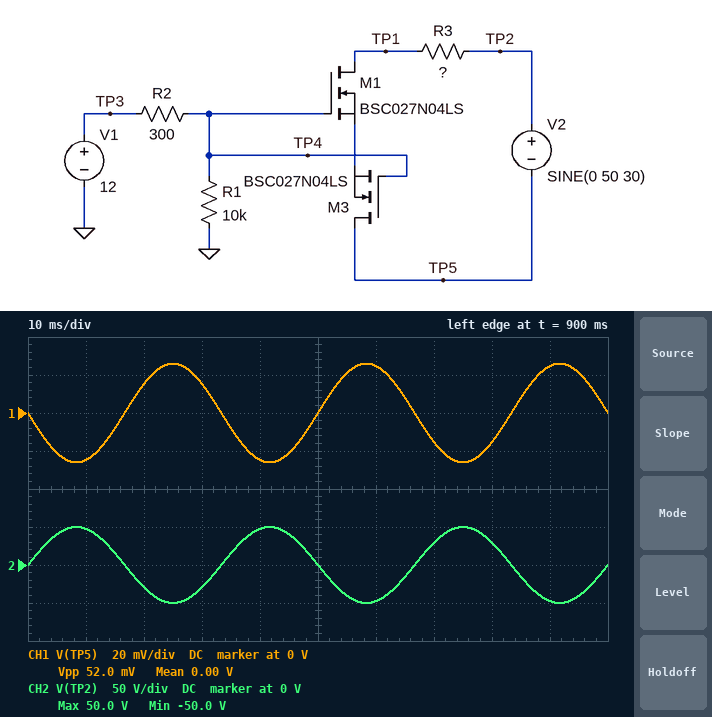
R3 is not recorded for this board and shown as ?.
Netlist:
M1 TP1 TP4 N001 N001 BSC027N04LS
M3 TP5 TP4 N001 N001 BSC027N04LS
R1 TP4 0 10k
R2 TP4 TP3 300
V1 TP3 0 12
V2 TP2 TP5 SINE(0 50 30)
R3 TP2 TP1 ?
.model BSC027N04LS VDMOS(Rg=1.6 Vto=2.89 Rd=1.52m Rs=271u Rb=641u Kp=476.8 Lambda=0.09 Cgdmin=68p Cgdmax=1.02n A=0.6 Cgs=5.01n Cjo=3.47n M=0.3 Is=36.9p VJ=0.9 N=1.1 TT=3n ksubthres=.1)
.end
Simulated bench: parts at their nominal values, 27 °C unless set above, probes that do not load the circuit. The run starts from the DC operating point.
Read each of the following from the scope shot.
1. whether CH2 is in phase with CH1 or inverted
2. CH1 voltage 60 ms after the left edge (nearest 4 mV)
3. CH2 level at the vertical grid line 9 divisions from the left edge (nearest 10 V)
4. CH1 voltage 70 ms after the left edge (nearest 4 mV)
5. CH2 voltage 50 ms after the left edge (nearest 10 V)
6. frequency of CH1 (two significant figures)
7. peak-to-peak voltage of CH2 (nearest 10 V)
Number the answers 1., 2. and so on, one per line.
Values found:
1. inverted
2. 24 mV
3. -50 V
4. -16 mV
5. 0 V
6. 30 Hz
7. 100 V
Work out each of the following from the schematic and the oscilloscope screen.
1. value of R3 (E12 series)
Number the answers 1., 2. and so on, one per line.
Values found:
1. 3.9 Ω
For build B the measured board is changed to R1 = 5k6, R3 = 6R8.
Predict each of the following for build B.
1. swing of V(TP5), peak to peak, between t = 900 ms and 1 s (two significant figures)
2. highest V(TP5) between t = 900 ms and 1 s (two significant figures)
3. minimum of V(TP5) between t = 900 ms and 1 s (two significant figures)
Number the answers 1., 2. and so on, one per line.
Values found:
1. 30 mV
2. 15 mV
3. -15 mV
